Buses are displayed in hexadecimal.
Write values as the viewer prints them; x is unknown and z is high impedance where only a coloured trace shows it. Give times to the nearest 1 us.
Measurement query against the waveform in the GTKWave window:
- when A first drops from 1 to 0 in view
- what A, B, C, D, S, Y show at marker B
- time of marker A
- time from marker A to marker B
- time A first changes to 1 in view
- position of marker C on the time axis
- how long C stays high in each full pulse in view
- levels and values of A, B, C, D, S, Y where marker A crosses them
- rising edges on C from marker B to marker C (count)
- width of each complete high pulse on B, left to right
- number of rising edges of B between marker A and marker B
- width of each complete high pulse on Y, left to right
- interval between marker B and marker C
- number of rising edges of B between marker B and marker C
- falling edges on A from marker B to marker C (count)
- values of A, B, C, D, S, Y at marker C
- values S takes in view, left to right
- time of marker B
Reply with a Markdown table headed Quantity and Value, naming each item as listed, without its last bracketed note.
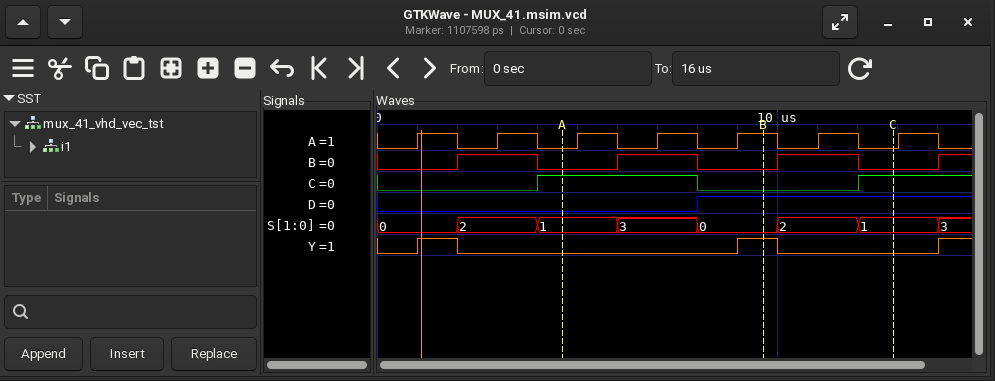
| Quantity | Value |
|---|---|
| when A first drops from 1 to 0 in view | 2 us |
| what A, B, C, D, S, Y show at marker B | A=1, B=0, C=0, D=1, S=0, Y=1 |
| time of marker A | 5 us |
| time from marker A to marker B | 5 us |
| time A first changes to 1 in view | 1 us |
| position of marker C on the time axis | 13 us |
| how long C stays high in each full pulse in view | 4 us |
| levels and values of A, B, C, D, S, Y where marker A crosses them | A=0, B=0, C=1, D=0, S=1, Y=0 |
| rising edges on C from marker B to marker C | 1 |
| width of each complete high pulse on B, left to right | 2 us, 2 us, 2 us |
| number of rising edges of B between marker A and marker B | 1 |
| width of each complete high pulse on Y, left to right | 1 us, 1 us |
| interval between marker B and marker C | 3 us |
| number of rising edges of B between marker B and marker C | 1 |
| falling edges on A from marker B to marker C | 2 |
| values of A, B, C, D, S, Y at marker C | A=0, B=0, C=1, D=1, S=1, Y=0 |
| values S takes in view, left to right | 0, 2, 1, 3, 0, 2, 1, 3 |
| time of marker B | 10 us |
